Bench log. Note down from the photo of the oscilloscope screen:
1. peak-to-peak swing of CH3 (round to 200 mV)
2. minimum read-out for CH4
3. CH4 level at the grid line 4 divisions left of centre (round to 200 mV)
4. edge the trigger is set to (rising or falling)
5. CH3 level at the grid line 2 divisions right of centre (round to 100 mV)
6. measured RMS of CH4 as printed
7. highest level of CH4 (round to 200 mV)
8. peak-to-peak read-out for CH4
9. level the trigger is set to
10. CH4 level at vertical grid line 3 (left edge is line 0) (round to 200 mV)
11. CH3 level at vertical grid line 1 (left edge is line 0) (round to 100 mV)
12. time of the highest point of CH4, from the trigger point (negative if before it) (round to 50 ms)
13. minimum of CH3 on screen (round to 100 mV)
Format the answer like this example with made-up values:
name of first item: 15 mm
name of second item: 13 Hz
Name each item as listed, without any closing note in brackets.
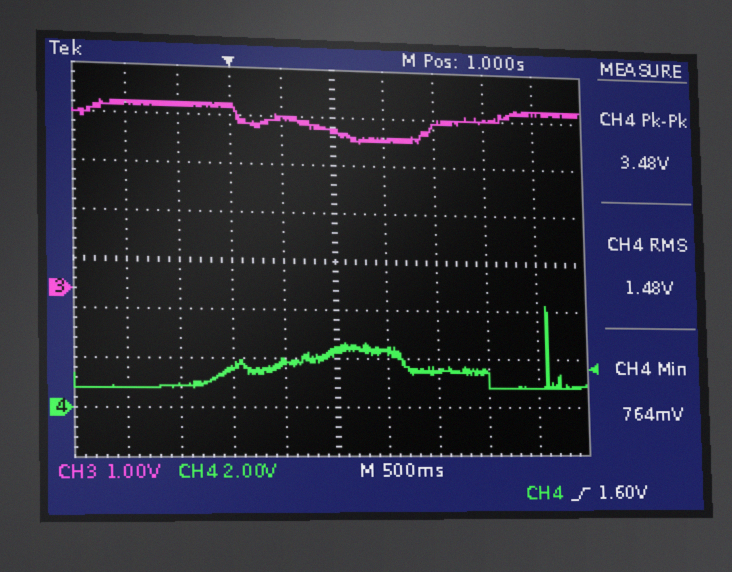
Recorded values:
peak-to-peak swing of CH3: 800 mV
minimum read-out for CH4: 764 mV
CH4 level at the grid line 4 divisions left of centre: 800 mV
edge the trigger is set to: rising
CH3 level at the grid line 2 divisions right of centre: 3.4 V
measured RMS of CH4 as printed: 1.48 V
highest level of CH4: 4.2 V
peak-to-peak read-out for CH4: 3.48 V
level the trigger is set to: 1.60 V
CH4 level at vertical grid line 3 (left edge is line 0): 1.6 V
CH3 level at vertical grid line 1 (left edge is line 0): 3.8 V
time of the highest point of CH4, from the trigger point (negative if before it): +3.10 s
minimum of CH3 on screen: 3.1 V
